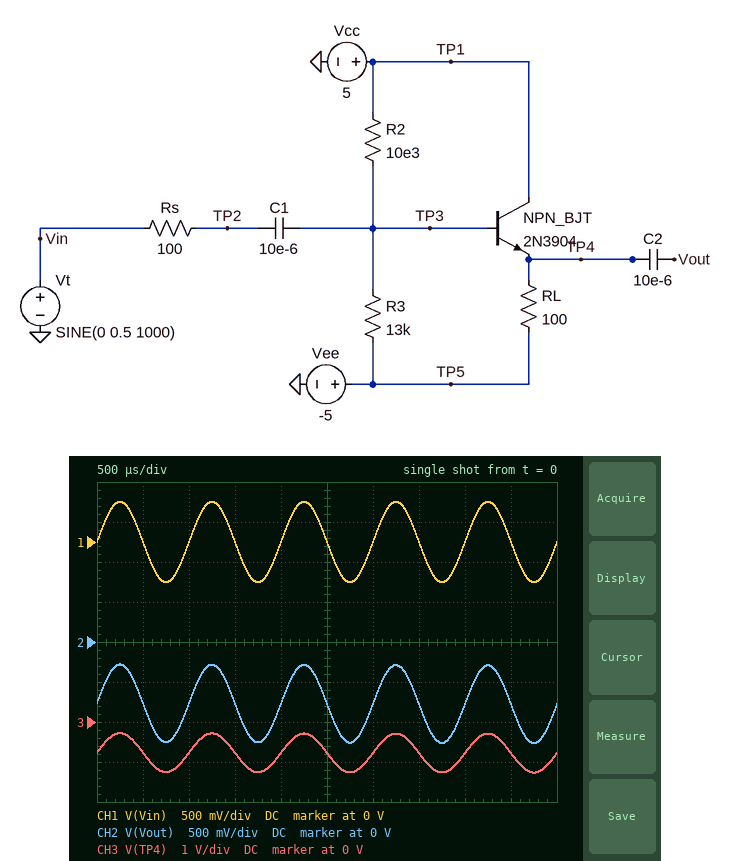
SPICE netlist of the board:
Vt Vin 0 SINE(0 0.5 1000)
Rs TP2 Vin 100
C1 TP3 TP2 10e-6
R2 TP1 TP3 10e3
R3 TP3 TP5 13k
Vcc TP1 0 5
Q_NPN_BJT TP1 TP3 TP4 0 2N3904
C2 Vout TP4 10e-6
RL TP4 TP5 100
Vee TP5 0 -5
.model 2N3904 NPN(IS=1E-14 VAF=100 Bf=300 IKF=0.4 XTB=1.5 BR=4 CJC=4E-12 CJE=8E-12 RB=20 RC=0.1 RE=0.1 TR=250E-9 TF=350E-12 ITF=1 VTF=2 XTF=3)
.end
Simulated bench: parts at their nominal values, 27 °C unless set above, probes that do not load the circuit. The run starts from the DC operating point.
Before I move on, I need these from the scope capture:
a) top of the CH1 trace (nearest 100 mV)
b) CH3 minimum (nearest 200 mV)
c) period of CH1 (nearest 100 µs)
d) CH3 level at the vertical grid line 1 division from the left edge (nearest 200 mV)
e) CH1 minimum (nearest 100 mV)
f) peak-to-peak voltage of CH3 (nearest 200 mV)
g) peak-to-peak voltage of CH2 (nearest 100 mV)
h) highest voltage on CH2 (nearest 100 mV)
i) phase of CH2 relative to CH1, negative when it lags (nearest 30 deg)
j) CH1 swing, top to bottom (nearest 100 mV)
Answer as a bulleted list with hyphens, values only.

- 500 mV
- -1.2 V
- 1.0 ms
- -800 mV
- -500 mV
- 1.0 V
- 1.0 V
- -300 mV
- 0 deg
- 1.0 V
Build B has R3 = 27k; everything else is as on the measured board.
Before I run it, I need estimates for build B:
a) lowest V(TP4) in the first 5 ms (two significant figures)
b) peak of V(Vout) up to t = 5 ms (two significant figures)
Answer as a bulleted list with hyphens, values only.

- -1.2 V
- -190 mV
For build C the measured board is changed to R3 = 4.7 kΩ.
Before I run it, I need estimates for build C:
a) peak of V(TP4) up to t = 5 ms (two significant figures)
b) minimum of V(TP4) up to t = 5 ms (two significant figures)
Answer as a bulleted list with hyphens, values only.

- -370 mV
- -1.6 V
